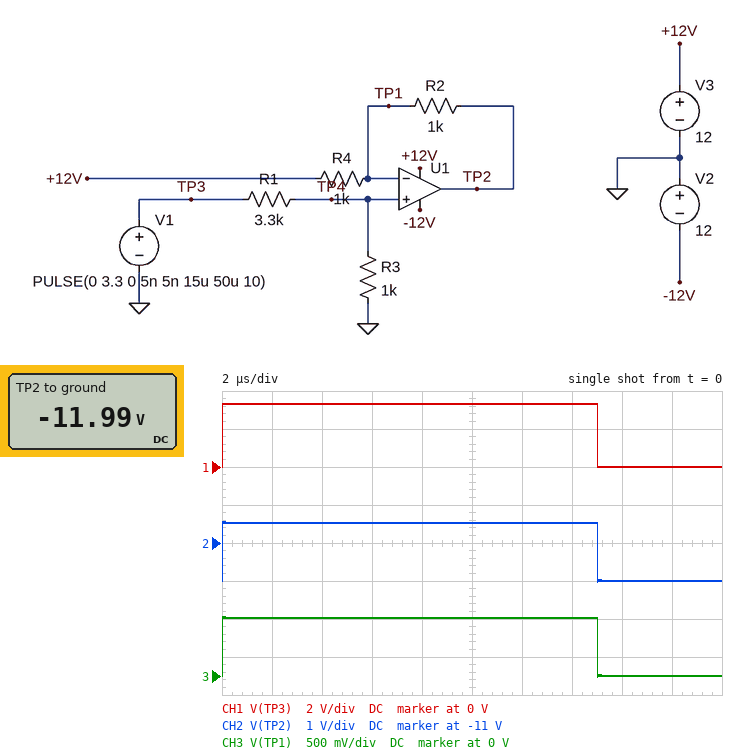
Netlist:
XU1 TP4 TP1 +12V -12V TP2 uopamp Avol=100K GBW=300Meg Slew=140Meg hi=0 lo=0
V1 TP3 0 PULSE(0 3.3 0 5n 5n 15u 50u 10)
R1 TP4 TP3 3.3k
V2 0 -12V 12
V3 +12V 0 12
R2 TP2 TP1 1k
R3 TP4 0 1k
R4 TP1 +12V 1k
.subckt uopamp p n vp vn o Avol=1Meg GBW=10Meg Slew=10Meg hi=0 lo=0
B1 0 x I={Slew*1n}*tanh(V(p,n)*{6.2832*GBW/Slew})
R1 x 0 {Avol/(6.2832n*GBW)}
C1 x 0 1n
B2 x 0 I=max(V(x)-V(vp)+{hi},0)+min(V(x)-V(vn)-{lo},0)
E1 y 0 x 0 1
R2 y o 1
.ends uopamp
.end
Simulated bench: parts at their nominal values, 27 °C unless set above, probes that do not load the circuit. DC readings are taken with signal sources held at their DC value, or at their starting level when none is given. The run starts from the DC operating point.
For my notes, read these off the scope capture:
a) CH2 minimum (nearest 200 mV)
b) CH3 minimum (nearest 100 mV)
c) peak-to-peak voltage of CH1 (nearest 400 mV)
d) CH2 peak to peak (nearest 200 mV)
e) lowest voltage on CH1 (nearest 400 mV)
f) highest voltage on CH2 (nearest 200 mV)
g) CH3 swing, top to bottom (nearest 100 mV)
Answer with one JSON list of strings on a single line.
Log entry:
["-12.0 V", "0 V", "3.2 V", "1.6 V", "0 V", "-10.4 V", "800 mV"]
